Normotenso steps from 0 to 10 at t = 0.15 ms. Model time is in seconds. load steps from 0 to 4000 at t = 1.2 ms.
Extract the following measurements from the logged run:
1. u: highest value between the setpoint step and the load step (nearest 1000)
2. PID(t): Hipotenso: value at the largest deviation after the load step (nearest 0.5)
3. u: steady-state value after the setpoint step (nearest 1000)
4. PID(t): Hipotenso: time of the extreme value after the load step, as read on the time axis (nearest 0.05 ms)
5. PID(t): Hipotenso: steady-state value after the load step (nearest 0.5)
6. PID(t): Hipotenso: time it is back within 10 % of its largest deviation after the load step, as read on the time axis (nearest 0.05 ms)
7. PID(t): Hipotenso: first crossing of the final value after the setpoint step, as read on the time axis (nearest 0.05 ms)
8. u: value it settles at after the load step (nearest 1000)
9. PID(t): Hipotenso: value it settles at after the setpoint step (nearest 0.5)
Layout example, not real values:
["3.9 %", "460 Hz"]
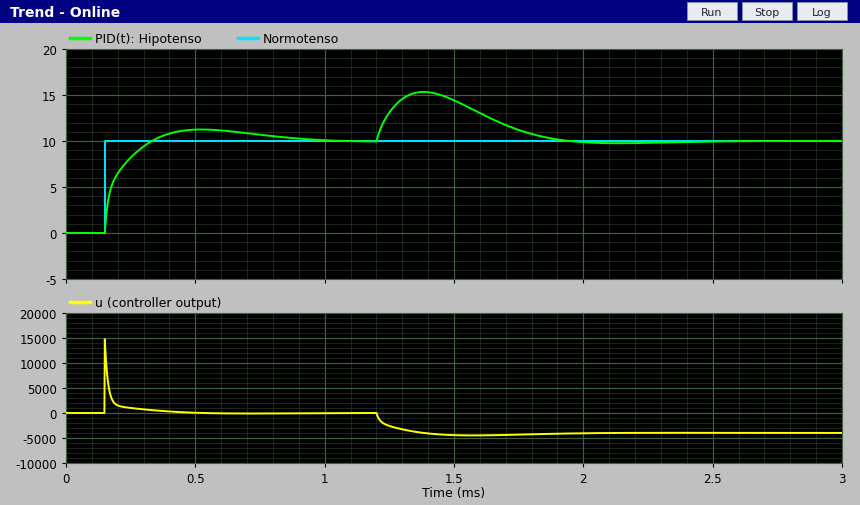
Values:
["15000", "15.5", "0", "1.40 ms", "10.0", "1.85 ms", "0.35 ms", "-4000", "10.0"]
